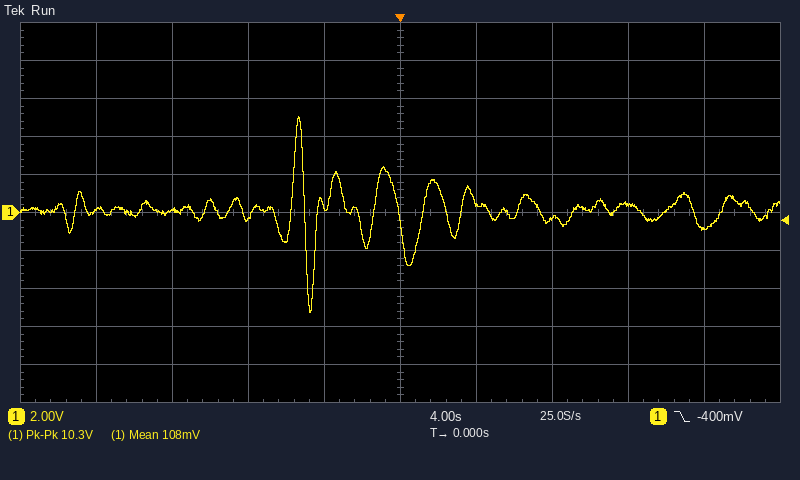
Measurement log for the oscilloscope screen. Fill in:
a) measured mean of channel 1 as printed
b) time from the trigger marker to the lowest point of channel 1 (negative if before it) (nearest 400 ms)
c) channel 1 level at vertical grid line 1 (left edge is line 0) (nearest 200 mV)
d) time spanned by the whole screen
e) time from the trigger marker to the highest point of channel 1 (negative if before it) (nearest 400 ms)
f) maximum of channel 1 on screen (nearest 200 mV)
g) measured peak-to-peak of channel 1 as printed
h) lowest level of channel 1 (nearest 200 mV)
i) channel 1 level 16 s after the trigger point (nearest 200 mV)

108 mV
-4.8 s
0.0 V
40 s
-5.2 s
5.0 V
10.3 V
-5.2 V
-800 mV
